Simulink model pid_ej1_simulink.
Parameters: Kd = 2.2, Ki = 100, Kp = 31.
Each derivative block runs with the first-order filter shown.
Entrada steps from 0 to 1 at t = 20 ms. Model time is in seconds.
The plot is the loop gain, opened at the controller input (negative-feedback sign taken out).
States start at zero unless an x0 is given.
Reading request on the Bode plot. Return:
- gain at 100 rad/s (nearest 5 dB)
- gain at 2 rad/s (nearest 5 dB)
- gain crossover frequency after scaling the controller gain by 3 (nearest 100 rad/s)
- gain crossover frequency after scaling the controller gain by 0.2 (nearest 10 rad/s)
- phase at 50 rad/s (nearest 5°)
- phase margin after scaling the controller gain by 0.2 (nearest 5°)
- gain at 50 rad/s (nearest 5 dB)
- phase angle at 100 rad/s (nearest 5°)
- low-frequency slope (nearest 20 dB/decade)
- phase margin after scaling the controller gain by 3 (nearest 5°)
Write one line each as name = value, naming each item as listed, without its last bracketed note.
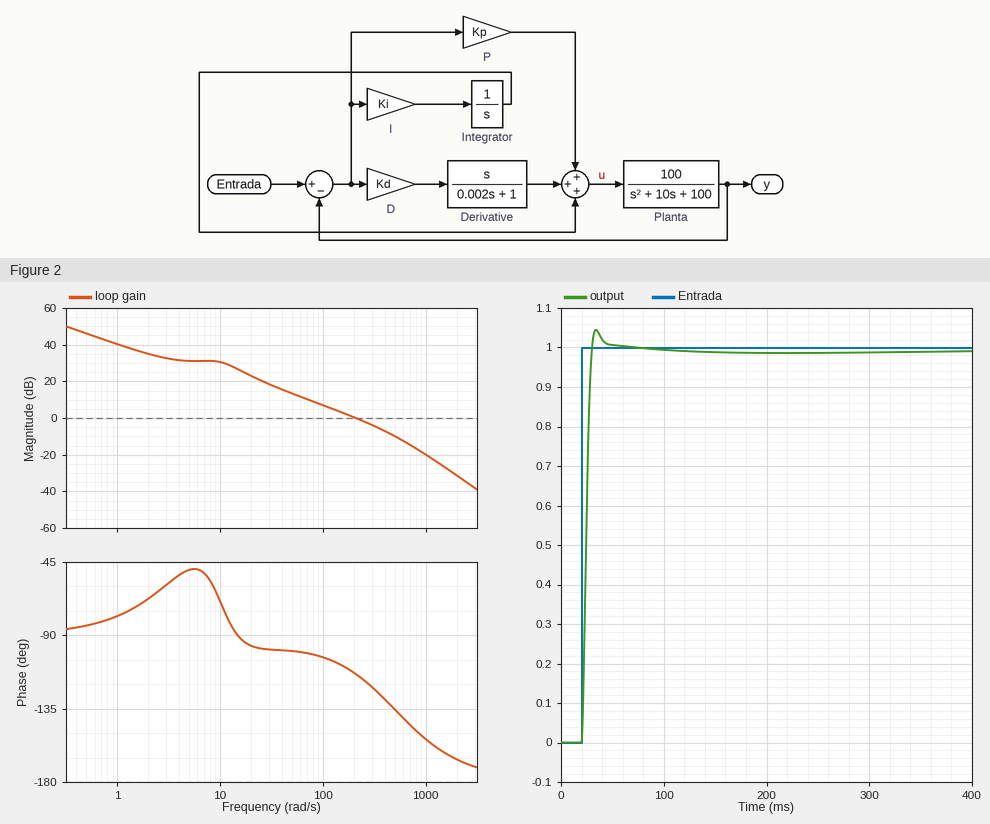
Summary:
gain at 100 rad/s = 5 dB
gain at 2 rad/s = 35 dB
gain crossover frequency after scaling the controller gain by 3 = 500 rad/s
gain crossover frequency after scaling the controller gain by 0.2 = 50 rad/s
phase at 50 rad/s = -100°
phase margin after scaling the controller gain by 0.2 = 80°
gain at 50 rad/s = 15 dB
phase angle at 100 rad/s = -105°
low-frequency slope = -20 dB/decade
phase margin after scaling the controller gain by 3 = 45°
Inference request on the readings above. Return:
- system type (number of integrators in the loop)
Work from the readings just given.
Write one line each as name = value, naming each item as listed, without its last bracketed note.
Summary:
system type = 1
